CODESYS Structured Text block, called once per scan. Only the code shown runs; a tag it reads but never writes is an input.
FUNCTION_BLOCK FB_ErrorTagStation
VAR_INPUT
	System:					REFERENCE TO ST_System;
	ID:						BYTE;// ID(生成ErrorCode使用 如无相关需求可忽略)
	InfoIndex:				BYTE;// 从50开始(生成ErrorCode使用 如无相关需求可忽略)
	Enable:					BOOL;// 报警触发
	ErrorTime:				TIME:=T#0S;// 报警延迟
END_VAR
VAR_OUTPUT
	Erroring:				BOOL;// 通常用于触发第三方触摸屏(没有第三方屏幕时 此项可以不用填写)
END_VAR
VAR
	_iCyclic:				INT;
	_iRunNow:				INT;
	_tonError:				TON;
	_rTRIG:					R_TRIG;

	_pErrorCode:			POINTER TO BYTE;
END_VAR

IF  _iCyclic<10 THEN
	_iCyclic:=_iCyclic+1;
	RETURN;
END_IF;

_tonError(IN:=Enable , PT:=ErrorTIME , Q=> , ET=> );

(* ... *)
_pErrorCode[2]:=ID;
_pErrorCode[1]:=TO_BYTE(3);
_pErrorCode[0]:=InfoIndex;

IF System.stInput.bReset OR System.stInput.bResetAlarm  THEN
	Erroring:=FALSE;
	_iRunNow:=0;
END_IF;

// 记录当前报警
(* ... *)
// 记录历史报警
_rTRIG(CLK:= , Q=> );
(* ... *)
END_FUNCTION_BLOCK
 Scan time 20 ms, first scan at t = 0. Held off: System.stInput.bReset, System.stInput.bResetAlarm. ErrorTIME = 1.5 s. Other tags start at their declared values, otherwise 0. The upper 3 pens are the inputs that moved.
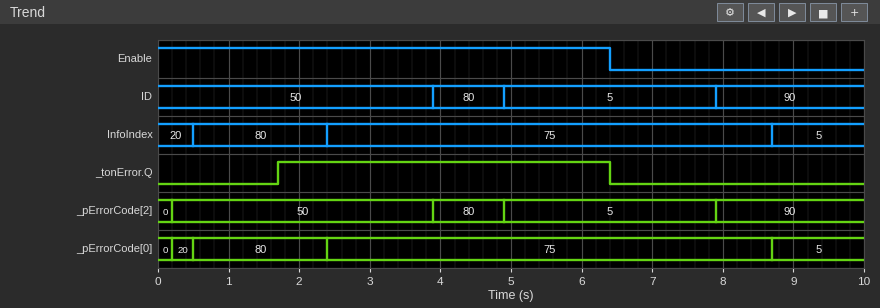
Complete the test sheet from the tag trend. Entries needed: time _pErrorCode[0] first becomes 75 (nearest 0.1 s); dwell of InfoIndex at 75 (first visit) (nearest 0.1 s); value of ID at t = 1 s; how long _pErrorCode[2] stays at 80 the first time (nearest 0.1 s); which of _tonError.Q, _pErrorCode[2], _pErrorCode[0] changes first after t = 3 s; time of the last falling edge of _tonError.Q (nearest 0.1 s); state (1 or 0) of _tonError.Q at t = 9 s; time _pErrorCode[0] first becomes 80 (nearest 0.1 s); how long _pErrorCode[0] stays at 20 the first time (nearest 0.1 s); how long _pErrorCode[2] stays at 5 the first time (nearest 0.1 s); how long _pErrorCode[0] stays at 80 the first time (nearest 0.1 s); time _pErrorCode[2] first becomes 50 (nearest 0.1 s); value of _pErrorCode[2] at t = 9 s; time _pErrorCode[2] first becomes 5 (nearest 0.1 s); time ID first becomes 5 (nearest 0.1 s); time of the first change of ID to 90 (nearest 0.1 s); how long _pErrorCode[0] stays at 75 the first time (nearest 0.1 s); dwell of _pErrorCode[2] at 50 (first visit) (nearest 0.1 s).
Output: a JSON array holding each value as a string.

["2.4 s", "6.3 s", "50", "1.0 s", "_pErrorCode[2]", "6.4 s", "0", "0.5 s", "0.3 s", "3.0 s", "1.9 s", "0.2 s", "90", "4.9 s", "4.9 s", "7.9 s", "6.3 s", "3.7 s"]
